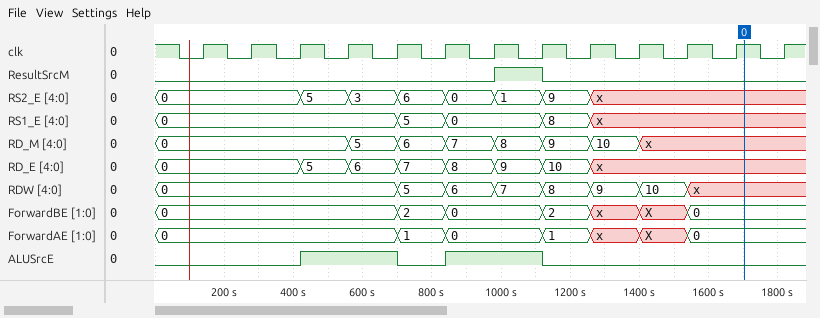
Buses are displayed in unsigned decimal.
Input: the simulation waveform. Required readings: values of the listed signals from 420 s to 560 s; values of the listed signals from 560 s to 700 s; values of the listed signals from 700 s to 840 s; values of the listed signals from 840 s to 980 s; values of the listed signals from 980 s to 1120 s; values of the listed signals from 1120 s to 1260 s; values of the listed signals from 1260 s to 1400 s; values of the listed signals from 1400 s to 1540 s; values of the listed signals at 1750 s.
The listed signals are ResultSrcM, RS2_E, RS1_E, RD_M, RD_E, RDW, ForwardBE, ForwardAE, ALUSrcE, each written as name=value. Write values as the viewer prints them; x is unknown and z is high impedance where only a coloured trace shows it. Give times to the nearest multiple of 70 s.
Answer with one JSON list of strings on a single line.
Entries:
["ResultSrcM=0, RS2_E=5, RS1_E=0, RD_M=0, RD_E=5, RDW=0, ForwardBE=0, ForwardAE=0, ALUSrcE=1", "ResultSrcM=0, RS2_E=3, RS1_E=0, RD_M=5, RD_E=6, RDW=0, ForwardBE=0, ForwardAE=0, ALUSrcE=1", "ResultSrcM=0, RS2_E=6, RS1_E=5, RD_M=6, RD_E=7, RDW=5, ForwardBE=2, ForwardAE=1, ALUSrcE=0", "ResultSrcM=0, RS2_E=0, RS1_E=0, RD_M=7, RD_E=8, RDW=6, ForwardBE=0, ForwardAE=0, ALUSrcE=1", "ResultSrcM=1, RS2_E=1, RS1_E=0, RD_M=8, RD_E=9, RDW=7, ForwardBE=0, ForwardAE=0, ALUSrcE=1", "ResultSrcM=0, RS2_E=9, RS1_E=8, RD_M=9, RD_E=10, RDW=8, ForwardBE=2, ForwardAE=1, ALUSrcE=0", "ResultSrcM=0, RS2_E=x, RS1_E=x, RD_M=10, RD_E=x, RDW=9, ForwardBE=x, ForwardAE=x, ALUSrcE=0", "ResultSrcM=0, RS2_E=x, RS1_E=x, RD_M=x, RD_E=x, RDW=10, ForwardBE=X, ForwardAE=X, ALUSrcE=0", "ResultSrcM=0, RS2_E=x, RS1_E=x, RD_M=x, RD_E=x, RDW=x, ForwardBE=0, ForwardAE=0, ALUSrcE=0"]
